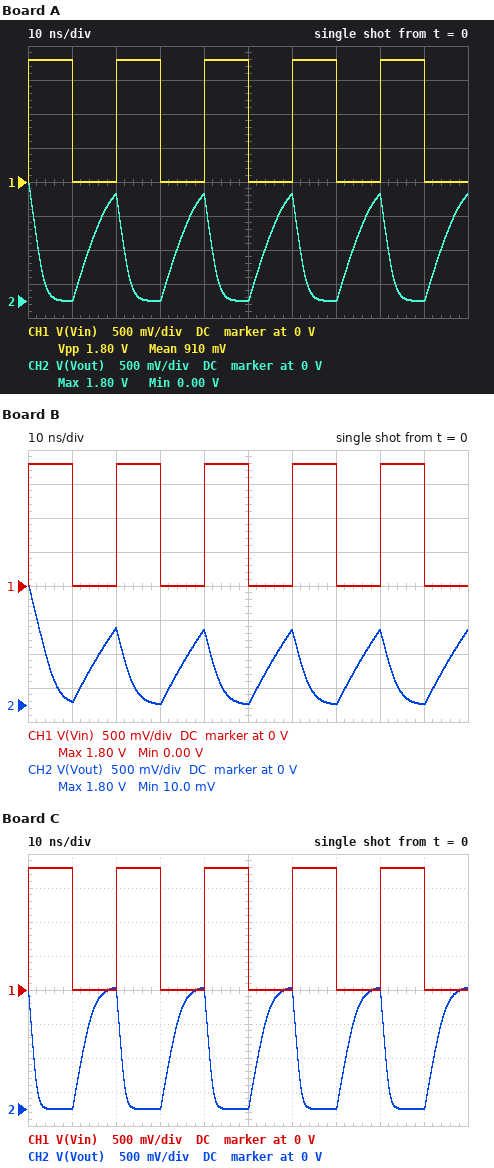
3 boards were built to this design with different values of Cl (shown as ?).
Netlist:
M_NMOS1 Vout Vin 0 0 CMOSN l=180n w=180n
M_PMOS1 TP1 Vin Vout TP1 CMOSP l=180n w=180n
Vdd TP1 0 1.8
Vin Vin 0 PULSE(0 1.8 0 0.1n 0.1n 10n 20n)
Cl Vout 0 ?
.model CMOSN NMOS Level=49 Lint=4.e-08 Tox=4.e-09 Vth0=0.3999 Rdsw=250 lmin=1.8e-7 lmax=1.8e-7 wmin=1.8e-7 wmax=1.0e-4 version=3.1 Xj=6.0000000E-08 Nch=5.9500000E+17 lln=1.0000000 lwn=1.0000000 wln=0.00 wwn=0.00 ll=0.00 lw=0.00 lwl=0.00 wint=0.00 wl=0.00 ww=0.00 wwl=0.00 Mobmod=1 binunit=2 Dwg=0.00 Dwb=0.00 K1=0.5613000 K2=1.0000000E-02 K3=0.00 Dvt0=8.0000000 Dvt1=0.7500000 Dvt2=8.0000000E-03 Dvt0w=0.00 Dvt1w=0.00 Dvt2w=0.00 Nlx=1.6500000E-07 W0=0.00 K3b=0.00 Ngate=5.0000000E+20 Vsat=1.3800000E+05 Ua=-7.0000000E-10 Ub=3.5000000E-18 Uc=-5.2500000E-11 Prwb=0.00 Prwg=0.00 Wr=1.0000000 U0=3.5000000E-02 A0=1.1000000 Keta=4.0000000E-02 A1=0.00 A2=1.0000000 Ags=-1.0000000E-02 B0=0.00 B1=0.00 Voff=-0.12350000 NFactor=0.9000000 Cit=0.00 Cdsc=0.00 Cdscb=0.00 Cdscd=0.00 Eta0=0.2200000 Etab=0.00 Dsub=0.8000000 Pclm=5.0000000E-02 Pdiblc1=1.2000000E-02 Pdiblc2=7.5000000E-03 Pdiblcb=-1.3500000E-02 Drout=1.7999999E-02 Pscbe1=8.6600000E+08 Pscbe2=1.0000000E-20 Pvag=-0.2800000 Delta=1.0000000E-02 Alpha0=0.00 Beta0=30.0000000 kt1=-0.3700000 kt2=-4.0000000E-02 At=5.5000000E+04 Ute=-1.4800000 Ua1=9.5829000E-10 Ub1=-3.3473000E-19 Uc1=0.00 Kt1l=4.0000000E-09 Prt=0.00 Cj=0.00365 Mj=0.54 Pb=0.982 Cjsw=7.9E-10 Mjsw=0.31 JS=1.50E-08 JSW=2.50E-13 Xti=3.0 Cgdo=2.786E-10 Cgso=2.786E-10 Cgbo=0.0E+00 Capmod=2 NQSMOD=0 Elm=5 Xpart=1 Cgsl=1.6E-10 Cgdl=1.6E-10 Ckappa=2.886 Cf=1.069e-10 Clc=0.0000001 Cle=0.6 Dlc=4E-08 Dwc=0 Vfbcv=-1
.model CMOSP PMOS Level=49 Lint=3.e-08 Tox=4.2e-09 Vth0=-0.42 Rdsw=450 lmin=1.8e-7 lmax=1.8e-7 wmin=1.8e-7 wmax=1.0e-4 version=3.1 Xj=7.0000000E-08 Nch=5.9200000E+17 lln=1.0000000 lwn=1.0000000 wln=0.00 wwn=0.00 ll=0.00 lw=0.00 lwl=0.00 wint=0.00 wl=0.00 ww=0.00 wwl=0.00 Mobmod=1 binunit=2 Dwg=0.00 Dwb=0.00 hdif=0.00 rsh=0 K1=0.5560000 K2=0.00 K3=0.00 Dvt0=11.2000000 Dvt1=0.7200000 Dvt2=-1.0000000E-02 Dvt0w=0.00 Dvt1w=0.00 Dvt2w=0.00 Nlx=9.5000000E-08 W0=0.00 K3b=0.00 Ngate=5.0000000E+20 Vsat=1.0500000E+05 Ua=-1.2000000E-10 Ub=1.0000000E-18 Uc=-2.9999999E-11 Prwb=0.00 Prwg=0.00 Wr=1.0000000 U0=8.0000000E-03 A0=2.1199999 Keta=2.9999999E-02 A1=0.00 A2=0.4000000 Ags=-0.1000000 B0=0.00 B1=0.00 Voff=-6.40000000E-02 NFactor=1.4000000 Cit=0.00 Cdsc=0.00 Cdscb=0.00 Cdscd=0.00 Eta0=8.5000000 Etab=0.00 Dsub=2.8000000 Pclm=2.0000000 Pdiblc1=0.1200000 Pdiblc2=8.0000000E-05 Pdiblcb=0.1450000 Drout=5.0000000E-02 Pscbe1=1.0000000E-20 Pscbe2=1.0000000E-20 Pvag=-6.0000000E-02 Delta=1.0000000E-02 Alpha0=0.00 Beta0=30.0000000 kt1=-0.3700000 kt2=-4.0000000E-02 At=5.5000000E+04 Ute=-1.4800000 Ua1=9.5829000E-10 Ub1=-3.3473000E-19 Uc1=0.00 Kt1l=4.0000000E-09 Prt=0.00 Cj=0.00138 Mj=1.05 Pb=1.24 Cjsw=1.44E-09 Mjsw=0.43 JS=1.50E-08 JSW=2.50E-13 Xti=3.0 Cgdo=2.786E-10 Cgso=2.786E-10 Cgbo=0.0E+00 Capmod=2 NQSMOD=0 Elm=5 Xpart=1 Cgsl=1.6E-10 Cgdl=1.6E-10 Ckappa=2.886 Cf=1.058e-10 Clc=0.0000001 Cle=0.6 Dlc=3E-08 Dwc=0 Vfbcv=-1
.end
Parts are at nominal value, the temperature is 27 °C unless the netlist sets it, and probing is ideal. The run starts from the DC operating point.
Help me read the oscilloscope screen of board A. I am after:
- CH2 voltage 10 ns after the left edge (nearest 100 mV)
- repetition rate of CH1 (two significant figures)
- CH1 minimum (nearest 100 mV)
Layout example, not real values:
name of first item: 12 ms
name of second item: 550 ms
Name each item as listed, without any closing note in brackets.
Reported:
CH2 voltage 10 ns after the left edge: 0 V
repetition rate of CH1: 50 MHz
CH1 minimum: 0 V
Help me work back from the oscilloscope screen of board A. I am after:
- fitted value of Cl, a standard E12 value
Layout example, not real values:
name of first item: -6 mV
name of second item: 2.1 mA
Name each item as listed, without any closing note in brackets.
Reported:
fitted value of Cl, a standard E12 value: 270 fF
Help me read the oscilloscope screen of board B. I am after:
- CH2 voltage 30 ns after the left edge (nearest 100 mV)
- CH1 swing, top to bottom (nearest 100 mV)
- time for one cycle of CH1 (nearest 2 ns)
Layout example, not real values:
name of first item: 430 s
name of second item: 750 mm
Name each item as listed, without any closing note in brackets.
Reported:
CH2 voltage 30 ns after the left edge: 0 V
CH1 swing, top to bottom: 1.8 V
time for one cycle of CH1: 20 ns
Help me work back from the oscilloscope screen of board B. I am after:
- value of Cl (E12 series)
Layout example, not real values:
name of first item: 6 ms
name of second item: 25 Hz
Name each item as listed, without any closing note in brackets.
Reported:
value of Cl: 470 fF
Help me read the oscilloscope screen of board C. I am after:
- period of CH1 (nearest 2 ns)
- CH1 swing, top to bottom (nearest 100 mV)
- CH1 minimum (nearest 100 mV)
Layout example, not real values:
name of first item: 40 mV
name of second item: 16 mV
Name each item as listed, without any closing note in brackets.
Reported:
period of CH1: 20 ns
CH1 swing, top to bottom: 1.8 V
CH1 minimum: 0 V
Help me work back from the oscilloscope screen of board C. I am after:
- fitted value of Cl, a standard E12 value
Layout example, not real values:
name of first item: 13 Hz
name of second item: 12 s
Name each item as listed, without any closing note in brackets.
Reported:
fitted value of Cl, a standard E12 value: 150 fF
